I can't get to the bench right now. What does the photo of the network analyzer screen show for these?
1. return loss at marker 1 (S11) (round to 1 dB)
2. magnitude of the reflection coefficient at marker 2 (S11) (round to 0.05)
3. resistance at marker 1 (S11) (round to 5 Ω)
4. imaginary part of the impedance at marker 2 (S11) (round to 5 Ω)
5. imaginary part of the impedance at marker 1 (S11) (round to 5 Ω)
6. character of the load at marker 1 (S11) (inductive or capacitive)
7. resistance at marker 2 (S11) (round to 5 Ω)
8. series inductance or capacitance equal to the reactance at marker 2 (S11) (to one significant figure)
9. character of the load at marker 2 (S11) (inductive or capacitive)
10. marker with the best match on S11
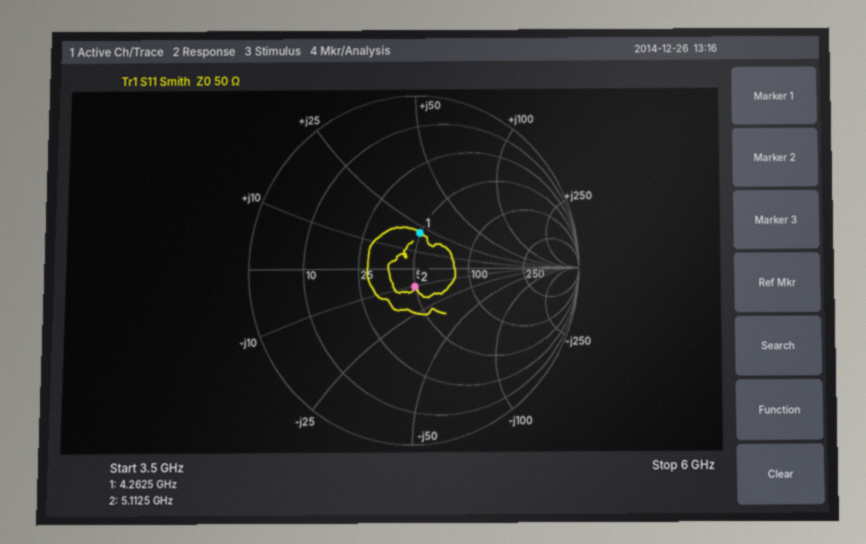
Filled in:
14 dB
0.10
50 Ω
-10 Ω
+20 Ω
inductive
50 Ω
3 pF
capacitive
marker 2
